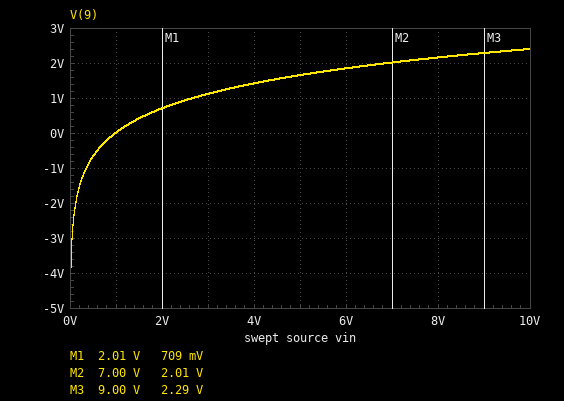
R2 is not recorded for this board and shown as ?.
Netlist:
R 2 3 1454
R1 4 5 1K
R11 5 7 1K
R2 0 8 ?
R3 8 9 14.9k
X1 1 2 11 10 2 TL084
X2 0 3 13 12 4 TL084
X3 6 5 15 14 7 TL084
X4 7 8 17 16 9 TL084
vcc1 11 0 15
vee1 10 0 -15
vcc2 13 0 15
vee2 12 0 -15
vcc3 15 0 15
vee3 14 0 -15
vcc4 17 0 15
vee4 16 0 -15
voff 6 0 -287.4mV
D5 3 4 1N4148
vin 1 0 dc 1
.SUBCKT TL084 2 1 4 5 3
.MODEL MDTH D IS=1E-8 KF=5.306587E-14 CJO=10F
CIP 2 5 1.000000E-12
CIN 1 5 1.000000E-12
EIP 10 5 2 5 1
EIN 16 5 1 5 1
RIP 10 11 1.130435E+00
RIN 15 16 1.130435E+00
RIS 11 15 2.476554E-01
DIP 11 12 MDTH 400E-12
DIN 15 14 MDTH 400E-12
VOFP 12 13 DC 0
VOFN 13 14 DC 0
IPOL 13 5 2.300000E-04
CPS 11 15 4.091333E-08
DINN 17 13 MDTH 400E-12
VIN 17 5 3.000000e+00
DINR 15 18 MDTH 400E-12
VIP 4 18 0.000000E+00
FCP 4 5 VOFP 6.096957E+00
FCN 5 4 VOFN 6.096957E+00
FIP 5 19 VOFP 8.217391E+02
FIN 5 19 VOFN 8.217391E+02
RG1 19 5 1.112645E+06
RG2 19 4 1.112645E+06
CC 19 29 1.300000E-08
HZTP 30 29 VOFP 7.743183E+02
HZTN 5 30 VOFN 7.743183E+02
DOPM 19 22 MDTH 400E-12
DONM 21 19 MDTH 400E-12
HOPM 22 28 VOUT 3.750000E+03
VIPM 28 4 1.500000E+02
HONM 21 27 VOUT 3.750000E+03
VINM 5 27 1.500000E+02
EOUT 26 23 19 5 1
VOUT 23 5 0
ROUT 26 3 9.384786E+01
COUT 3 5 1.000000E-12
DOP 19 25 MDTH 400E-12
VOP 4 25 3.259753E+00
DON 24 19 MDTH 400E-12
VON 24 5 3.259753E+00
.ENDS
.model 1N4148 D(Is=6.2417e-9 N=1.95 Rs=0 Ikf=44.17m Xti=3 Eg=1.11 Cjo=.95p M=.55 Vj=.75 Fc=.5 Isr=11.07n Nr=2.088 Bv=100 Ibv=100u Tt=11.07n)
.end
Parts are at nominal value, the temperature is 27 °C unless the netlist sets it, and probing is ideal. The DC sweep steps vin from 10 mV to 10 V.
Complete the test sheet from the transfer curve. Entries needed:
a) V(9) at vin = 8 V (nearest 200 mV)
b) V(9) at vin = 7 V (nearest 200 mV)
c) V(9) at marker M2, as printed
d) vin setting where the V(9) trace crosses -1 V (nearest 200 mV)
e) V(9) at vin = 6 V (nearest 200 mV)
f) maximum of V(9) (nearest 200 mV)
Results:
2.2 V
2.0 V
2.01 V
400 mV
1.8 V
2.4 V
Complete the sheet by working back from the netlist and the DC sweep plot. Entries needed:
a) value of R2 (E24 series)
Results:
910 Ω
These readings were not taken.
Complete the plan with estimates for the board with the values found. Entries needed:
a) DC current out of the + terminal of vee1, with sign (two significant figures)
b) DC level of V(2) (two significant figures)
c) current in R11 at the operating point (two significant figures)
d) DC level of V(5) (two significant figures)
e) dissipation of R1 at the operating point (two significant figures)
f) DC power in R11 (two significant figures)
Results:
-730 µA
1.0 V
290 µA
-290 mV
83 µW
83 µW
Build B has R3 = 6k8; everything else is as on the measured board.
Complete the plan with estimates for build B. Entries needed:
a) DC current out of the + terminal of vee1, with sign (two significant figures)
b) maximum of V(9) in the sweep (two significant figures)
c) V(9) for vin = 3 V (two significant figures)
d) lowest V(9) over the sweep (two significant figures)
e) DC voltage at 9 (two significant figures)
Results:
-730 µA
1.2 V
550 mV
-2.1 V
5.8 mV
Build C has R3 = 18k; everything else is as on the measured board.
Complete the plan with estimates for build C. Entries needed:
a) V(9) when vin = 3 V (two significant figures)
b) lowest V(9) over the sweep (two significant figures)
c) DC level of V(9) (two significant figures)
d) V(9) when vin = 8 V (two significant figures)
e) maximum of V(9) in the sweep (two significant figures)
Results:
1.3 V
-5.2 V
14 mV
2.6 V
2.9 V
